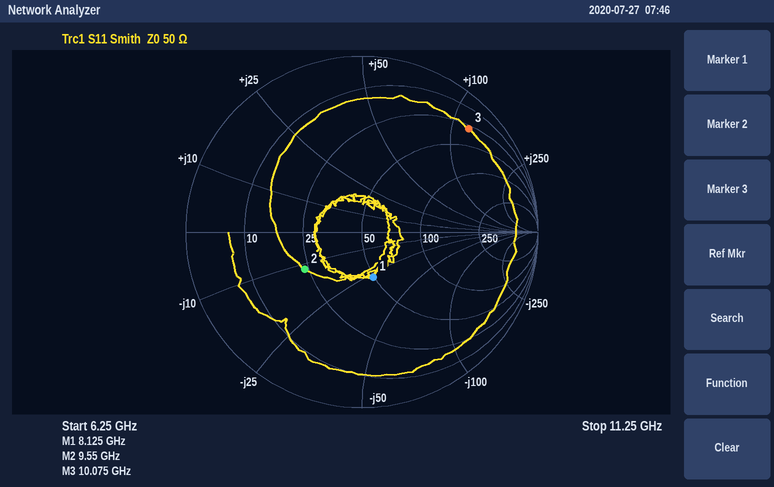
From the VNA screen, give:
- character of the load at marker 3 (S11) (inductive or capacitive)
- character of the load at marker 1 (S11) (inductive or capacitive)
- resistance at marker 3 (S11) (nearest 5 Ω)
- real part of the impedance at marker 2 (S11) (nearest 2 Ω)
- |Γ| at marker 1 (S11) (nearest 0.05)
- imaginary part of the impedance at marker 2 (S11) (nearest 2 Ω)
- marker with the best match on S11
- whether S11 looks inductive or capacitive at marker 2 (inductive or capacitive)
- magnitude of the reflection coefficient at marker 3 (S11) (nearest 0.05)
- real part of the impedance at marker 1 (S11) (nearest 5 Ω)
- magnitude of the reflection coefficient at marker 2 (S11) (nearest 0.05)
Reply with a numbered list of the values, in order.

1. inductive
2. capacitive
3. 30 Ω
4. 24 Ω
5. 0.25
6. -12 Ω
7. marker 1
8. capacitive
9. 0.85
10. 50 Ω
11. 0.40
